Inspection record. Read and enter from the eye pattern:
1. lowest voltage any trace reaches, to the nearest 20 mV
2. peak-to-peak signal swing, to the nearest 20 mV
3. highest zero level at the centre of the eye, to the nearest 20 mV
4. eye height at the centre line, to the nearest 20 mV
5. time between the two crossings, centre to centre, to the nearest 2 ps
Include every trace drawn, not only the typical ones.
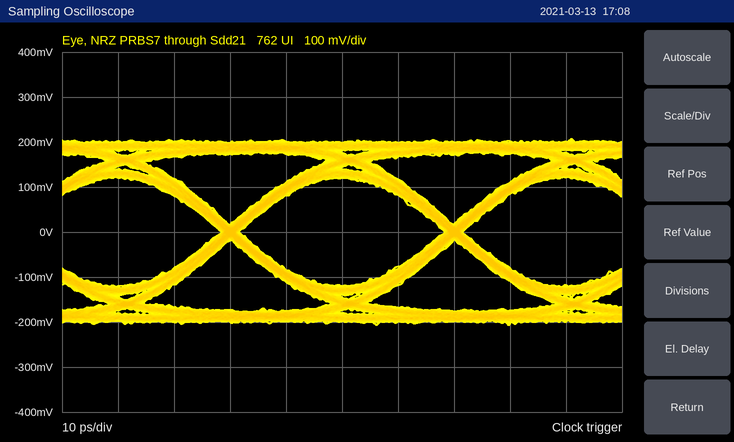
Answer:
-200 mV
420 mV
-120 mV
240 mV
40 ps
